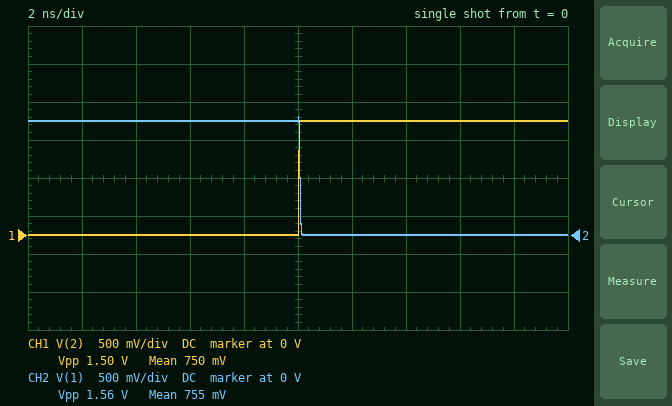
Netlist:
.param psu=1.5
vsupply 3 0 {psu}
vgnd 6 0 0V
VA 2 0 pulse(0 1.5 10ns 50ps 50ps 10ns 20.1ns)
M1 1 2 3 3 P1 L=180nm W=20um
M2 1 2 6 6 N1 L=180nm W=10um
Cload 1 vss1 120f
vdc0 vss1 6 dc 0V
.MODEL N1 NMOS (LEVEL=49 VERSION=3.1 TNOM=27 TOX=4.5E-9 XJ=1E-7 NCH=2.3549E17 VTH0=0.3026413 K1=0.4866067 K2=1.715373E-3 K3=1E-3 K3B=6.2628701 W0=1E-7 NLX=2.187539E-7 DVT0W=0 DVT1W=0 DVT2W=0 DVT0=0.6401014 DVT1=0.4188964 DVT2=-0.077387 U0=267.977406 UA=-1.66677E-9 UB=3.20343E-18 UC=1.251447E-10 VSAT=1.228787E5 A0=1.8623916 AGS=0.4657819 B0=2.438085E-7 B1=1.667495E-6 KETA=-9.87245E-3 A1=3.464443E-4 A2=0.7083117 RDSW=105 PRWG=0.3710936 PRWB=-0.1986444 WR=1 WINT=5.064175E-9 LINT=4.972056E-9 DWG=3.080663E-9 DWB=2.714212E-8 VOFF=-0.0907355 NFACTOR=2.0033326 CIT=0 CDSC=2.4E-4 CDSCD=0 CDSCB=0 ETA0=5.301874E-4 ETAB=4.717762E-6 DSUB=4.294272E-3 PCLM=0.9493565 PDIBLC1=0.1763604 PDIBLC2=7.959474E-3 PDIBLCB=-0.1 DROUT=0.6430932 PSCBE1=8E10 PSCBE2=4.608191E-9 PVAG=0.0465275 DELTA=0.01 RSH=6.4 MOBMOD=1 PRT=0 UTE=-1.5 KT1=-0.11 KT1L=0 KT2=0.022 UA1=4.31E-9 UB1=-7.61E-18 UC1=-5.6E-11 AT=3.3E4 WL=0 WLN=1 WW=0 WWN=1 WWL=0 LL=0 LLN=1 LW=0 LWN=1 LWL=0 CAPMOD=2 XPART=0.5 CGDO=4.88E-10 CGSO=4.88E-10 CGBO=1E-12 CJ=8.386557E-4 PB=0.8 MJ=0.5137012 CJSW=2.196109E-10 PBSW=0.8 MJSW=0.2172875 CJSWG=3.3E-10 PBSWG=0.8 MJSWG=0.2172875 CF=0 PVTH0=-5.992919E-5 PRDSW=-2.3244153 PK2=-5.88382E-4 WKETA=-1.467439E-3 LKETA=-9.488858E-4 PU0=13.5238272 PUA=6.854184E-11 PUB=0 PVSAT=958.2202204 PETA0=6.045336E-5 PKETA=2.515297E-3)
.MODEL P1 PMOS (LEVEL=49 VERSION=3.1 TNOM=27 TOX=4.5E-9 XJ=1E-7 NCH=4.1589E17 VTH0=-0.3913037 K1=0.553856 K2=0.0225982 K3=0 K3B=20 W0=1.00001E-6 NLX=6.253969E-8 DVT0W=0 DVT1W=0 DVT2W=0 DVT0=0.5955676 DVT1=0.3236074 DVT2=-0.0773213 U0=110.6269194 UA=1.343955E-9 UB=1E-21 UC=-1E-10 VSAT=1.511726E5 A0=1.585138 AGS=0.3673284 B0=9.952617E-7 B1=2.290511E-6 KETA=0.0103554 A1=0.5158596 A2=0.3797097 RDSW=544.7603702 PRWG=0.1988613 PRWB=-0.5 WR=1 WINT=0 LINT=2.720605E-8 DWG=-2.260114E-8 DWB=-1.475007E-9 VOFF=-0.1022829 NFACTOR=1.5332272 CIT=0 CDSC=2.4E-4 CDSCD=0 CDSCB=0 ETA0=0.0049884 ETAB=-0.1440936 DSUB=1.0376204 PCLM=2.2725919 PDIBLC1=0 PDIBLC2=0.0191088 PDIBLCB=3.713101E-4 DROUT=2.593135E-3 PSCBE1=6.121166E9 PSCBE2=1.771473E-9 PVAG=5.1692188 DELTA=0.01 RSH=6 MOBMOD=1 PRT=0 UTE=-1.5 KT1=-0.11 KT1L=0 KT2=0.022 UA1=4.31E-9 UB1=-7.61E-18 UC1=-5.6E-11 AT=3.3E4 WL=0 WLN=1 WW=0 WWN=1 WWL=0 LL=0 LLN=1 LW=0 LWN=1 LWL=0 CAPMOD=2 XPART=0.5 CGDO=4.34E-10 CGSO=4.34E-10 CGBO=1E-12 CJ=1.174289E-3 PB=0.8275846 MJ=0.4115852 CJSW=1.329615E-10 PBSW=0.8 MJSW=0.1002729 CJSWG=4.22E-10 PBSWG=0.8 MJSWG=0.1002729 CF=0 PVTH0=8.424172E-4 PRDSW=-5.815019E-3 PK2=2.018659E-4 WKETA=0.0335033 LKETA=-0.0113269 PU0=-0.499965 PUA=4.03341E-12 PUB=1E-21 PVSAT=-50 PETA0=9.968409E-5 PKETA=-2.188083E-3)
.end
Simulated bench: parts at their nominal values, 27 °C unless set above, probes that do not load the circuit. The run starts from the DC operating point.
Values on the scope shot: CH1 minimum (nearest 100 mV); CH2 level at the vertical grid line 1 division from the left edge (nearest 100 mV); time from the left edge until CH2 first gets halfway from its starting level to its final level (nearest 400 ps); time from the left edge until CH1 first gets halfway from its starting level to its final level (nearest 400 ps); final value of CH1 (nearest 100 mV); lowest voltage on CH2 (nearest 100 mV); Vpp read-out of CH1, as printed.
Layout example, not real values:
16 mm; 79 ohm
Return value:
0 V; 1.5 V; 10.0 ns; 10.0 ns; 1.5 V; 0 V; 1.50 V
